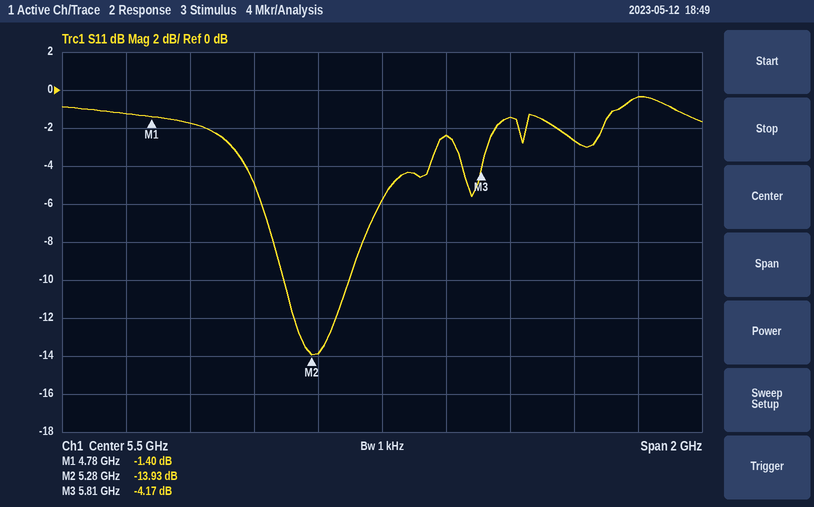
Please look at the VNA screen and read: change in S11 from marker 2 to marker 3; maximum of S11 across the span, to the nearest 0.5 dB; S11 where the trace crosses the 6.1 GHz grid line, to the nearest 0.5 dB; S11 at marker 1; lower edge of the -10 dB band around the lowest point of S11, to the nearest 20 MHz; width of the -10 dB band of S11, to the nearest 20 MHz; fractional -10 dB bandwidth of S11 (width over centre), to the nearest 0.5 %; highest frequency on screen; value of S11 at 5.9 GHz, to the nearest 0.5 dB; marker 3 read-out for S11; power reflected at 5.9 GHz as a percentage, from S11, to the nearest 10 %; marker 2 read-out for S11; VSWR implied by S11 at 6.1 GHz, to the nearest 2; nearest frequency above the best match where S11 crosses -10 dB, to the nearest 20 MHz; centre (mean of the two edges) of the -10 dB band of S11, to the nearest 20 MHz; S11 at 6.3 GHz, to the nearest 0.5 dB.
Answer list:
9.76 dB
-0.5 dB
-2.5 dB
-1.40 dB
5.20 GHz
200 MHz
4.0 %
6.5 GHz
-1.5 dB
-4.17 dB
70 %
-13.93 dB
6
5.40 GHz
5.30 GHz
-0.5 dB
